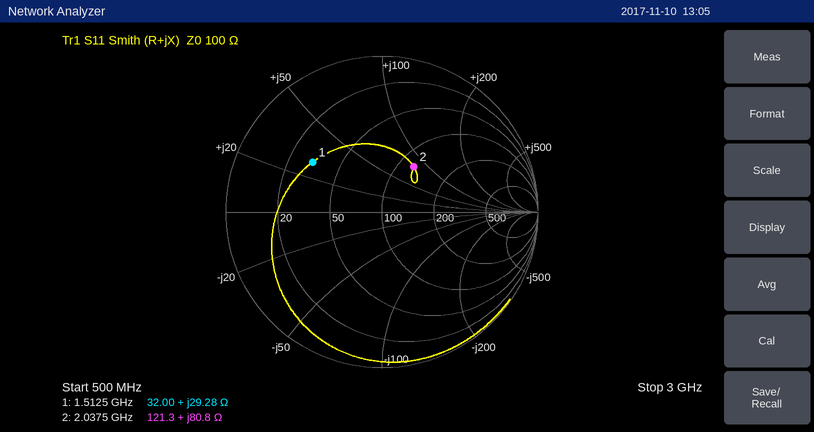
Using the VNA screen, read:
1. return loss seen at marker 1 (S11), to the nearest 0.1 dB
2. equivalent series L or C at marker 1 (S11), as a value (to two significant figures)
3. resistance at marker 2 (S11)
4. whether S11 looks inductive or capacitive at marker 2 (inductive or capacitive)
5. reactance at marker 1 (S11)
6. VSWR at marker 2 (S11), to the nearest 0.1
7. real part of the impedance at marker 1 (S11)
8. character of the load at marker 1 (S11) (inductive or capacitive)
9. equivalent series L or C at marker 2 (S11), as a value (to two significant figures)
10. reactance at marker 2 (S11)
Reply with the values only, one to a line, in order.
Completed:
5.2 dB
3.1 nH
121.3 Ω
inductive
+29.28 Ω
2.1
32.00 Ω
inductive
6.3 nH
+80.8 Ω
